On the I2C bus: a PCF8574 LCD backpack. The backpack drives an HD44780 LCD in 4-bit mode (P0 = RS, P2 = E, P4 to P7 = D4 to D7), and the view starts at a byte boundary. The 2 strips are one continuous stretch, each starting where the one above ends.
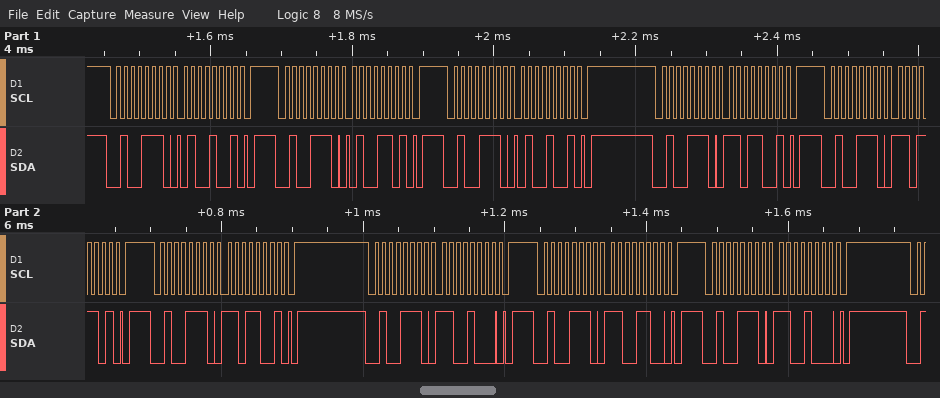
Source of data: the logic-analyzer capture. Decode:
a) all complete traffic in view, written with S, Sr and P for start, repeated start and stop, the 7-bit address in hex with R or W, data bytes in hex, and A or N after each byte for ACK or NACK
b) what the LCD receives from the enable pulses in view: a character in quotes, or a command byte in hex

S 27W A 49 A P S 27W A 4D A P S 27W A 49 A P S 27W A D9 A P S 27W A DD A P S 27W A D9 A P S 27W A C8 A P S 27W A CC A P S 27W A C8 A P
'M'
